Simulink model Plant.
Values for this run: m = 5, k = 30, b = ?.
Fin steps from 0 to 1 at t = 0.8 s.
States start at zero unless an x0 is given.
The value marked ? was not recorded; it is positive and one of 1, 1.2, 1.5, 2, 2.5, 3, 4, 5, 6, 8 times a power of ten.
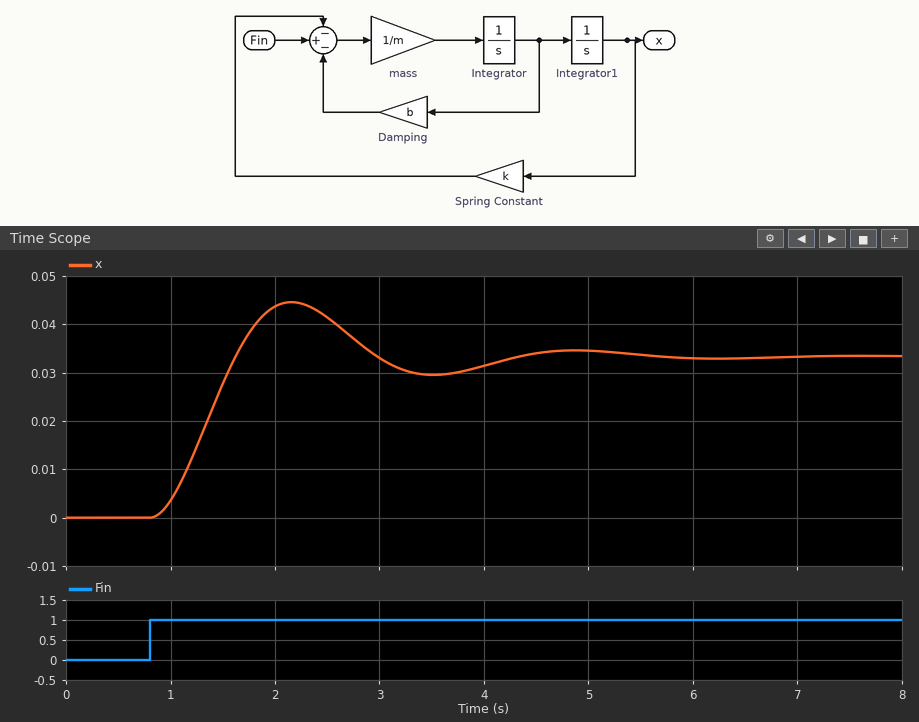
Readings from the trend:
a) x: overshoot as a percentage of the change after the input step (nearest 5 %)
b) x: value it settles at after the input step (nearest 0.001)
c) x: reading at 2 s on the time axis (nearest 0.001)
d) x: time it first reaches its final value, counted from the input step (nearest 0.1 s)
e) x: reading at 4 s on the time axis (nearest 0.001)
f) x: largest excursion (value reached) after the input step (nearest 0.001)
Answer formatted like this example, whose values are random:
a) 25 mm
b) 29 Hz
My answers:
a) 35 %
b) 0.033
c) 0.044
d) 0.8 s
e) 0.031
f) 0.045
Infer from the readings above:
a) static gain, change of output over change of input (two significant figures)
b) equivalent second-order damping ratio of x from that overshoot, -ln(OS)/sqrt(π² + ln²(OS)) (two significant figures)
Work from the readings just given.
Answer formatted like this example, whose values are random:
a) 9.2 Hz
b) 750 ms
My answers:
a) 0.033
b) 0.32
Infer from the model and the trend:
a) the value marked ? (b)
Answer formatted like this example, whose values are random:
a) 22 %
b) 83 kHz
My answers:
a) 8
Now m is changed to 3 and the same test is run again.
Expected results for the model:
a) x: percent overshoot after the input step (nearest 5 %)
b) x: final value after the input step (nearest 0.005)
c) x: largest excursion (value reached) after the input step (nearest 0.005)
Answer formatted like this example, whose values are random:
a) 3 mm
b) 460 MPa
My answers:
a) 25 %
b) 0.035
c) 0.040
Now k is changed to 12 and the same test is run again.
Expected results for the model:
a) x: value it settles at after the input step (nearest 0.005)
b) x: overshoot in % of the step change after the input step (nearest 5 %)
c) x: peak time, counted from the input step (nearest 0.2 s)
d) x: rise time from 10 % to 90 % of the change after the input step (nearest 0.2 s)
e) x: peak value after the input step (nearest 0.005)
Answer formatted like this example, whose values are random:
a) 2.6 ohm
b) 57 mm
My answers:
a) 0.085
b) 15 %
c) 2.4 s
d) 1.0 s
e) 0.095
